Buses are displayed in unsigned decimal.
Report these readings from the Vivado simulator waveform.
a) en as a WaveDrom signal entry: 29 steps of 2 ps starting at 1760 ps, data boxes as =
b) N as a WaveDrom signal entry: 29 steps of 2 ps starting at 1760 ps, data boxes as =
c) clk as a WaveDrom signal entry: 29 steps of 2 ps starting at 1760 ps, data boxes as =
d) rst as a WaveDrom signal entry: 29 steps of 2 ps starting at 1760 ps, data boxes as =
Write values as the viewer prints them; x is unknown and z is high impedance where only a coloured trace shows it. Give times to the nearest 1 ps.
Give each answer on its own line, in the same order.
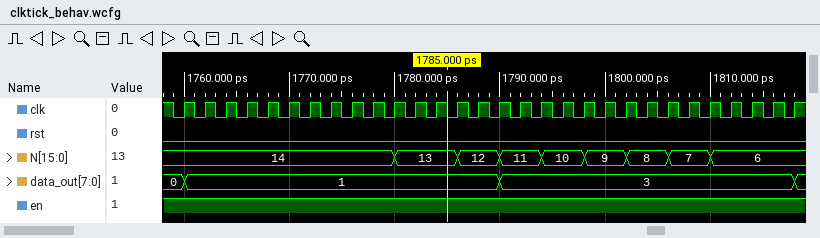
{name: 'en', wave: '1............................'}
{name: 'N', wave: '=.........=..=.=.=.=.=.=.=...', data: '14 13 12 11 10 9 8 7 6'}
{name: 'clk', wave: 'p............................'}
{name: 'rst', wave: '0............................'}
